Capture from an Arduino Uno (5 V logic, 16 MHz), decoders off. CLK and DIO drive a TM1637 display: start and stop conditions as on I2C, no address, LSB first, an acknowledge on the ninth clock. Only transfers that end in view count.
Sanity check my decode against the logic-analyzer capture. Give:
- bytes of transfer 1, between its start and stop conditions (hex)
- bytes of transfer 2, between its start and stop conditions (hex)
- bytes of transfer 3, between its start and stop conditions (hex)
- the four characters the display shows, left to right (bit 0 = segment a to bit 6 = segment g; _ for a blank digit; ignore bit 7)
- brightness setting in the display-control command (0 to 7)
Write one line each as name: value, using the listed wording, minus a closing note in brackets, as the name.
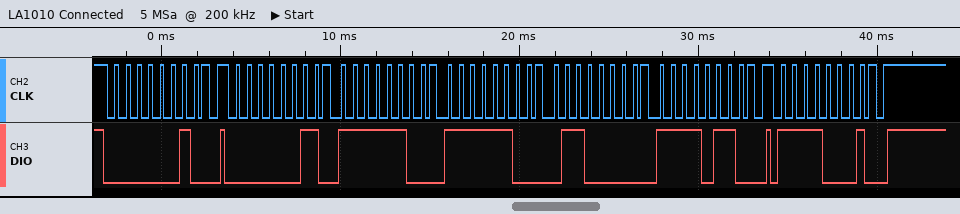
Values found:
bytes of transfer 1, between its start and stop conditions: 40
bytes of transfer 2, between its start and stop conditions: C0 3F 3F 06 6F
bytes of transfer 3, between its start and stop conditions: 8F
the four characters the display shows, left to right: 0019
brightness setting in the display-control command: 7
